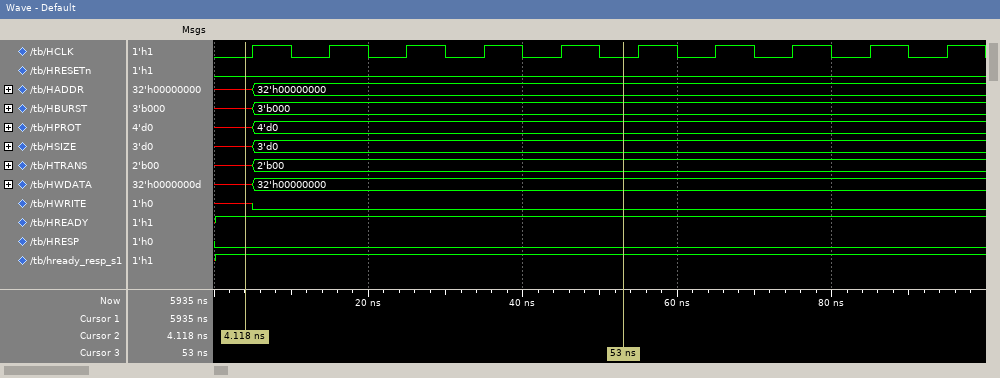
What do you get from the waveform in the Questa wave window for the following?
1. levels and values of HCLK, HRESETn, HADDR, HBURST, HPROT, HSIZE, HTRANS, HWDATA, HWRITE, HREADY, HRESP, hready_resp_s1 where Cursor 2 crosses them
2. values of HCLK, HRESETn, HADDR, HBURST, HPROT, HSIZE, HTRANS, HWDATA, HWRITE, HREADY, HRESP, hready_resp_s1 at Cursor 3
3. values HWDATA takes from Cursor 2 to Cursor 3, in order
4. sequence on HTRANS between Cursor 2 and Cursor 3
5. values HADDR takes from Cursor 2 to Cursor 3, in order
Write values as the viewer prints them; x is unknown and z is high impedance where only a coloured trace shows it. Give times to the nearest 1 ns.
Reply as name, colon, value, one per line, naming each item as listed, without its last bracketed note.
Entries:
levels and values of HCLK, HRESETn, HADDR, HBURST, HPROT, HSIZE, HTRANS, HWDATA, HWRITE, HREADY, HRESP, hready_resp_s1 where Cursor 2 crosses them: HCLK=0, HRESETn=0, HADDR=x, HBURST=x, HPROT=x, HSIZE=x, HTRANS=x, HWDATA=x, HWRITE=x, HREADY=1, HRESP=0, hready_resp_s1=1
values of HCLK, HRESETn, HADDR, HBURST, HPROT, HSIZE, HTRANS, HWDATA, HWRITE, HREADY, HRESP, hready_resp_s1 at Cursor 3: HCLK=0, HRESETn=0, HADDR=32'h00000000, HBURST=3'b000, HPROT=4'd0, HSIZE=3'd0, HTRANS=2'b00, HWDATA=32'h00000000, HWRITE=0, HREADY=1, HRESP=0, hready_resp_s1=1
values HWDATA takes from Cursor 2 to Cursor 3, in order: x, 32'h00000000
sequence on HTRANS between Cursor 2 and Cursor 3: x, 2'b00
values HADDR takes from Cursor 2 to Cursor 3, in order: x, 32'h00000000
